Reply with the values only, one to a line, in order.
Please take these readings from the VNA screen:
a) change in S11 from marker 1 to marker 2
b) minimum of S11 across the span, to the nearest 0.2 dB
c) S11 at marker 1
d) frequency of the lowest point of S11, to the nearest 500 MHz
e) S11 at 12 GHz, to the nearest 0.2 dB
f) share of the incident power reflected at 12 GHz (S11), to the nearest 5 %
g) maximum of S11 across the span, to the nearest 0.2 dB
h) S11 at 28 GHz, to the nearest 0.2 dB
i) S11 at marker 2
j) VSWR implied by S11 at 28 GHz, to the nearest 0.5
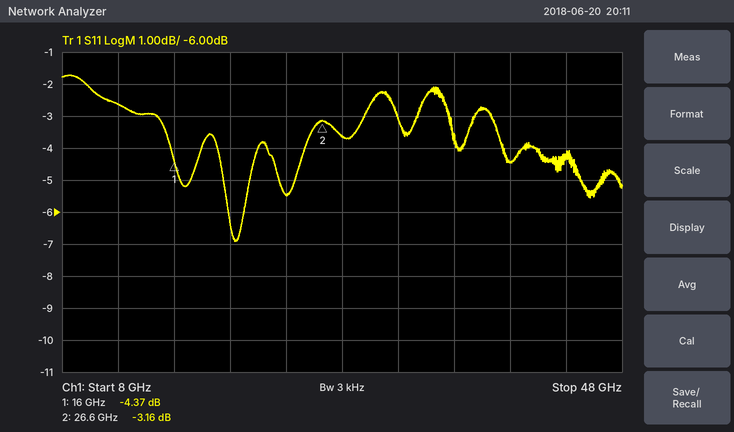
1.21 dB
-7.0 dB
-4.37 dB
20.5 GHz
-2.6 dB
55 %
-1.8 dB
-3.6 dB
-3.16 dB
5.0
